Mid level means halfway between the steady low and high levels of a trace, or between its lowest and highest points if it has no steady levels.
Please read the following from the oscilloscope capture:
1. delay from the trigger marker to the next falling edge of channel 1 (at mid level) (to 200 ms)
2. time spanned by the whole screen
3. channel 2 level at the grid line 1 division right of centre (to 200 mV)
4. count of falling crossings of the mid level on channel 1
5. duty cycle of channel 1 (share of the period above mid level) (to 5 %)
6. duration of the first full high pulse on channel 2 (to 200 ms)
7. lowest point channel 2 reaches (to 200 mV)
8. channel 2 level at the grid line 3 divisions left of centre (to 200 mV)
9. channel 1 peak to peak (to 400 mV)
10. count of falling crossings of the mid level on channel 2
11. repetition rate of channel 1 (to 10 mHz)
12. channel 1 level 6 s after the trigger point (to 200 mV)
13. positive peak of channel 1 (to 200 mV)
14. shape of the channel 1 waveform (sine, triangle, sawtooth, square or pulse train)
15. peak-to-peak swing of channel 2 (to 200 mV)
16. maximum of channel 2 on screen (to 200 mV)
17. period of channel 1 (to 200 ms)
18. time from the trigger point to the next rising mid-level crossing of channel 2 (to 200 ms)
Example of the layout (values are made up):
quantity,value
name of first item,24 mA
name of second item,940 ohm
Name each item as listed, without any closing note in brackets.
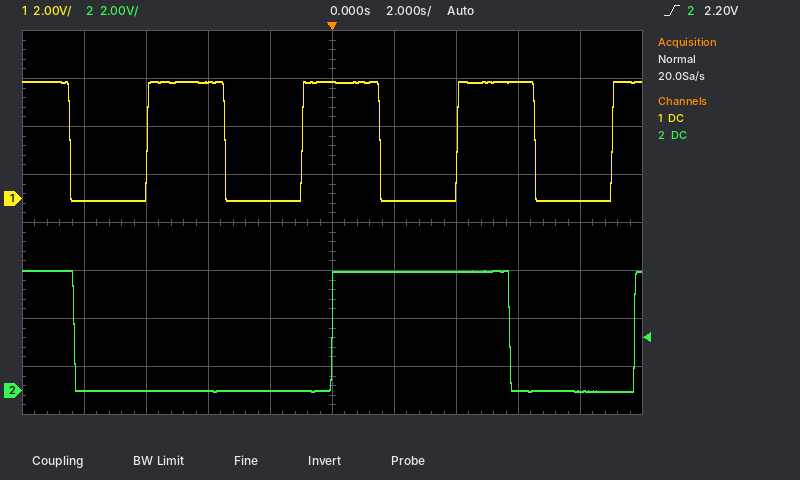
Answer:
quantity,value
delay from the trigger marker to the next falling edge of channel 1 (at mid level),1.6 s
time spanned by the whole screen,20 s
channel 2 level at the grid line 1 division right of centre,5.0 V
count of falling crossings of the mid level on channel 1,4
duty cycle of channel 1 (share of the period above mid level),50 %
duration of the first full high pulse on channel 2,5.8 s
lowest point channel 2 reaches,0.0 V
channel 2 level at the grid line 3 divisions left of centre,0.0 V
channel 1 peak to peak,4.8 V
count of falling crossings of the mid level on channel 2,2
repetition rate of channel 1,200 mHz
channel 1 level 6 s after the trigger point,4.8 V
positive peak of channel 1,4.8 V
shape of the channel 1 waveform,square
peak-to-peak swing of channel 2,5.0 V
maximum of channel 2 on screen,5.0 V
period of channel 1,5.0 s
time from the trigger point to the next rising mid-level crossing of channel 2,9.8 s
